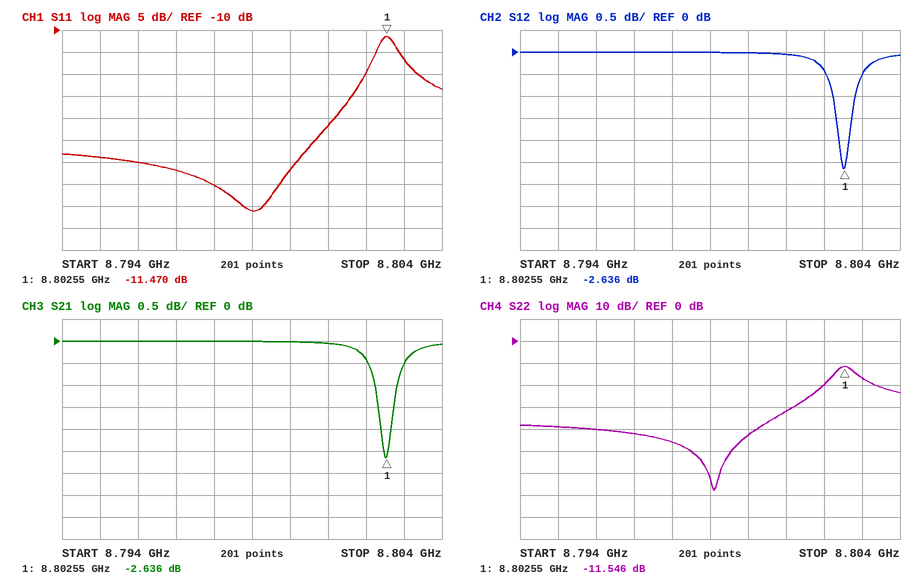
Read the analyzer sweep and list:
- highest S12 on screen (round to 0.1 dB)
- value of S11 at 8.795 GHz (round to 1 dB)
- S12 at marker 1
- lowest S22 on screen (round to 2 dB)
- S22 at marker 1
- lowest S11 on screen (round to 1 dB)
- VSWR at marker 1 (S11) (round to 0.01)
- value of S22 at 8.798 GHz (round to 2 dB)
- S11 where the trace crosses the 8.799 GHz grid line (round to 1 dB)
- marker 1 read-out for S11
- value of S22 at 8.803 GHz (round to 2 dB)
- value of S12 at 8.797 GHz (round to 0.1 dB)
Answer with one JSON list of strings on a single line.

["0.0 dB", "-39 dB", "-2.636 dB", "-68 dB", "-11.546 dB", "-51 dB", "1.73", "-46 dB", "-51 dB", "-11.470 dB", "-16 dB", "0.0 dB"]
